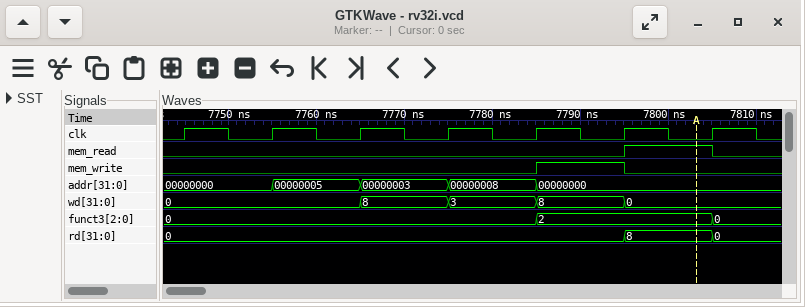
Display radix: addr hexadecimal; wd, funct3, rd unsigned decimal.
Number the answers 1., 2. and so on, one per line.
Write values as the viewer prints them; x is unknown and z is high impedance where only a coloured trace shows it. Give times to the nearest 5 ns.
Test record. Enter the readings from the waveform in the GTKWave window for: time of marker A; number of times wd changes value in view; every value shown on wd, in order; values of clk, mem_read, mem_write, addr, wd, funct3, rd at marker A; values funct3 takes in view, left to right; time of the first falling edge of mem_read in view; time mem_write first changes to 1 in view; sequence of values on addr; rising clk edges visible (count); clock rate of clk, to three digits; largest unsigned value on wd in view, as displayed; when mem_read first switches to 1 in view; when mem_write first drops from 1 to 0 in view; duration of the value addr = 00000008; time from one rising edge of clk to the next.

1. 7805 ns
2. 4
3. 0, 8, 3, 8, 0
4. clk=0, mem_read=1, mem_write=0, addr=00000000, wd=0, funct3=2, rd=8
5. 0, 2, 0
6. 7805 ns
7. 7785 ns
8. 00000000, 00000005, 00000003, 00000008, 00000000
9. 7
10. 100 MHz
11. 8
12. 7795 ns
13. 7795 ns
14. 10 ns
15. 10 ns
